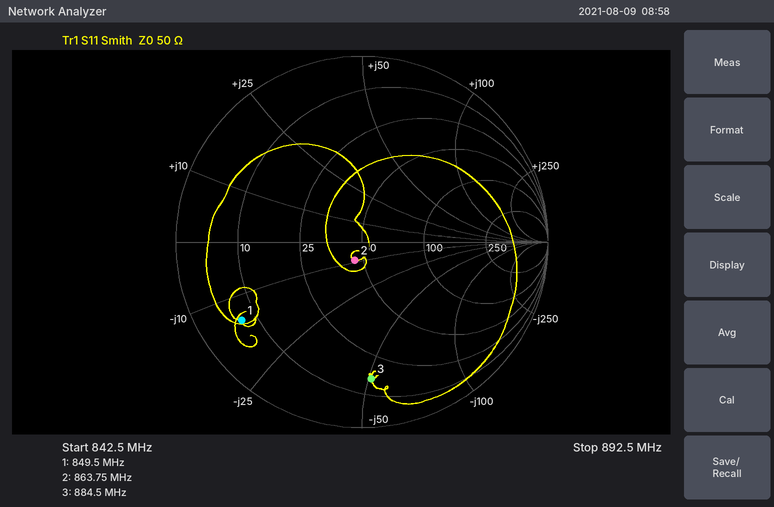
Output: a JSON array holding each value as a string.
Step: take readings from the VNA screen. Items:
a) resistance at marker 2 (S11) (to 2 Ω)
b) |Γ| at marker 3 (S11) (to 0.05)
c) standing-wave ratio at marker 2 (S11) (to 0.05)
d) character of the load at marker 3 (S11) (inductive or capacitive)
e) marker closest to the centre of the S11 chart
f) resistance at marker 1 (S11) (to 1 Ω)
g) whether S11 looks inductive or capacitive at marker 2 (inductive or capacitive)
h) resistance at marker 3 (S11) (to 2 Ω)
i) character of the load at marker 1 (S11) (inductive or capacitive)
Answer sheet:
["46 Ω", "0.75", "1.25", "capacitive", "marker 2", "7 Ω", "capacitive", "16 Ω", "capacitive"]
